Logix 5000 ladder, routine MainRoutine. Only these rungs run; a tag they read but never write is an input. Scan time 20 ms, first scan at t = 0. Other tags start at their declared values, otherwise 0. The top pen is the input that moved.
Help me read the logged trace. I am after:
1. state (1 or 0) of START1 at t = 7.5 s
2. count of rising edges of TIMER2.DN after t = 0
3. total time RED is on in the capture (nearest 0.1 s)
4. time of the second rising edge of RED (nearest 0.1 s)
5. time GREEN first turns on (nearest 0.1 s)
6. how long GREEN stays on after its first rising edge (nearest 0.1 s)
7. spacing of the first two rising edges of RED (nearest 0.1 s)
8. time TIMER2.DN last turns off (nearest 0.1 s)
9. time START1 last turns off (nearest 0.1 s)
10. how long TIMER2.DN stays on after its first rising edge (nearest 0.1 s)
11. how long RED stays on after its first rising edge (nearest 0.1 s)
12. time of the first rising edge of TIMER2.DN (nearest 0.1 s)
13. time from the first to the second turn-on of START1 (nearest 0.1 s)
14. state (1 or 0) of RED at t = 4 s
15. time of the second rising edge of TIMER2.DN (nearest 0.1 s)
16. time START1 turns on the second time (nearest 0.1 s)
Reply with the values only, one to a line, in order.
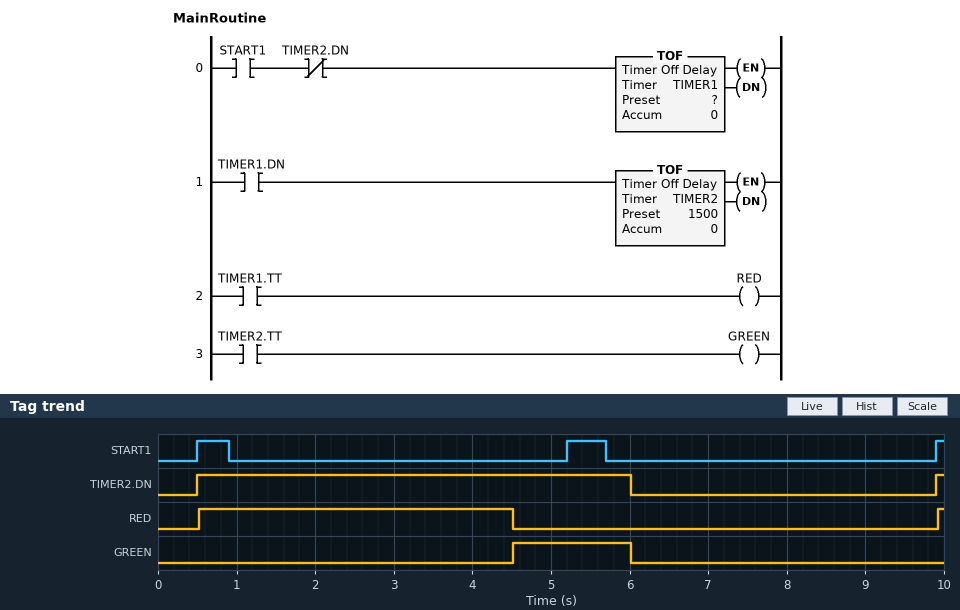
0
2
4.1 s
9.9 s
4.5 s
1.5 s
9.4 s
6.0 s
5.7 s
5.5 s
4.0 s
0.5 s
4.7 s
1
9.9 s
5.2 s
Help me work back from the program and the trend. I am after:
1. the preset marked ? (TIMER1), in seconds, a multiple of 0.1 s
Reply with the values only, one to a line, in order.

4.0 s
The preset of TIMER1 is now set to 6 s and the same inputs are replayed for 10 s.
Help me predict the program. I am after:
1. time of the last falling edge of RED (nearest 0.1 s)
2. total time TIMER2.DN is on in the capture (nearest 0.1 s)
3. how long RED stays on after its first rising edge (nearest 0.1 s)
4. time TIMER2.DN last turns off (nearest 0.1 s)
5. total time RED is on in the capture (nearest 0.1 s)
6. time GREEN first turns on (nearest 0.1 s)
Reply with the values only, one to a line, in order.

6.5 s
7.6 s
6.0 s
8.0 s
6.1 s
6.5 s
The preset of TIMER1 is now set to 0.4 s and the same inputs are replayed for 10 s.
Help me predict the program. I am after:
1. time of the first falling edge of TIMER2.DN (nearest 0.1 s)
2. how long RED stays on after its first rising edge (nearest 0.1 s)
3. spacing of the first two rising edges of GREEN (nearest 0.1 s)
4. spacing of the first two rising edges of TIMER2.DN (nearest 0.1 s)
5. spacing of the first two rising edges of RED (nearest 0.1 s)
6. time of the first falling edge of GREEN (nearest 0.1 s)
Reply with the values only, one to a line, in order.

2.4 s
0.4 s
4.7 s
4.7 s
4.7 s
2.4 s
